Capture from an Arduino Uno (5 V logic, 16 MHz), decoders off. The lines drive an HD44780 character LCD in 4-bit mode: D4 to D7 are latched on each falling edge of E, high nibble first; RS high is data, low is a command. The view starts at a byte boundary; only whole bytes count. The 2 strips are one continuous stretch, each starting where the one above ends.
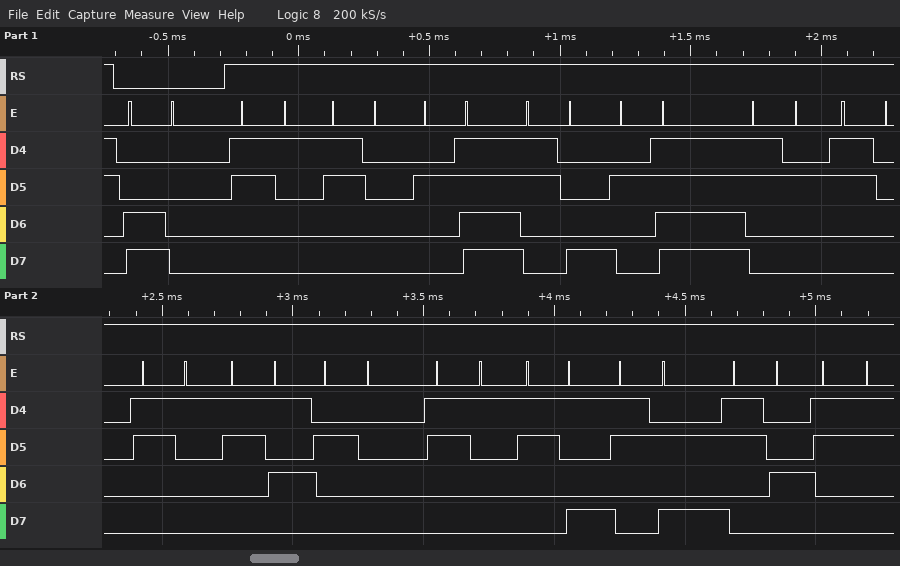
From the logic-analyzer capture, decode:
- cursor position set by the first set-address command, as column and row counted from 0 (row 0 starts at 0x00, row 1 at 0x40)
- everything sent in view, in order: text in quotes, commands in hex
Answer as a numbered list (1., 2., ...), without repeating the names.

1. column 0, row 1
2. 0xC0 "10/8/2015 19:43"
